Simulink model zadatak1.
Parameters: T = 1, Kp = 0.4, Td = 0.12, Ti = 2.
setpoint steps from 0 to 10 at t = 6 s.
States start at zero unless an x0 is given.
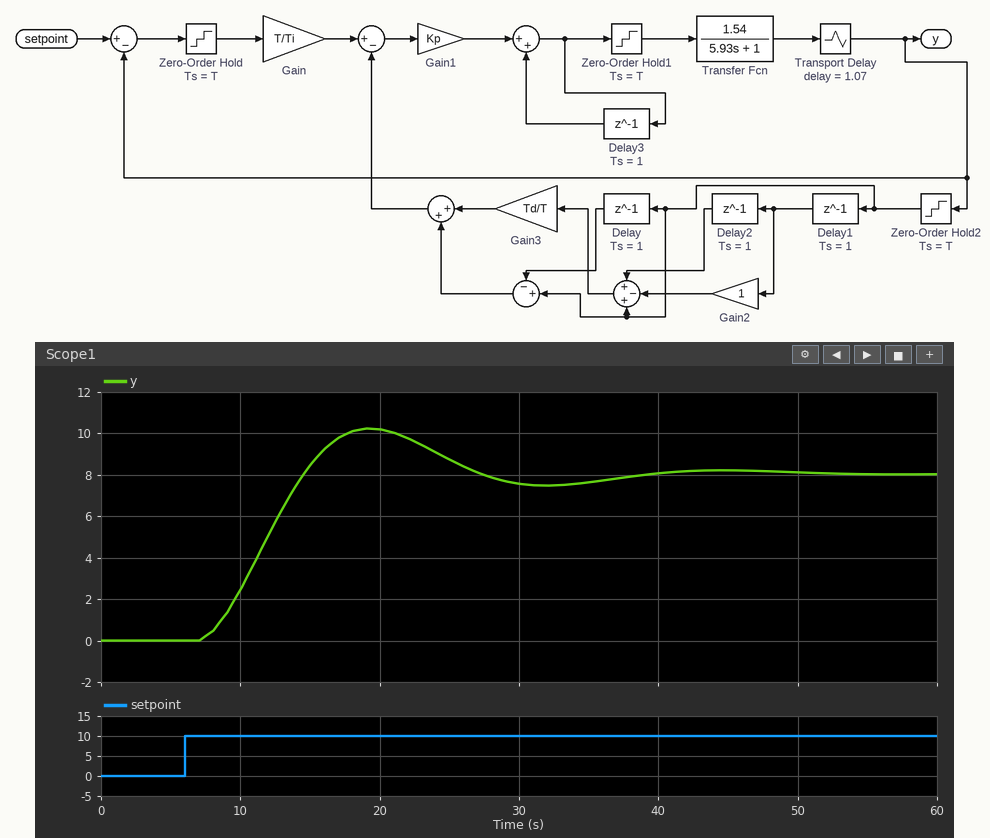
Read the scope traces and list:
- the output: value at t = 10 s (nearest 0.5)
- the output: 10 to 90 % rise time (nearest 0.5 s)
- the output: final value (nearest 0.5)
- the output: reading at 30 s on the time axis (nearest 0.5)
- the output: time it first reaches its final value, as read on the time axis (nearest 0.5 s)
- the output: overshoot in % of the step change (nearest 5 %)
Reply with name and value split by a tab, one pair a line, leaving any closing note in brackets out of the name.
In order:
the output: value at t = 10 s	2.5
the output: 10 to 90 % rise time	5.5 s
the output: final value	8.0
the output: reading at 30 s on the time axis	7.5
the output: time it first reaches its final value, as read on the time axis	14.5 s
the output: overshoot in % of the step change	25 %
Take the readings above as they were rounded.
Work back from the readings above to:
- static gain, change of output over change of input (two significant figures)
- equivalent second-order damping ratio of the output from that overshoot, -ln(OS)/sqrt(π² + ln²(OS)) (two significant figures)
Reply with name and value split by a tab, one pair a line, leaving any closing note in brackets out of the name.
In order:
static gain, change of output over change of input	0.80
equivalent second-order damping ratio of the output from that overshoot, -ln(OS)/sqrt(π² + ln²(OS))	0.40
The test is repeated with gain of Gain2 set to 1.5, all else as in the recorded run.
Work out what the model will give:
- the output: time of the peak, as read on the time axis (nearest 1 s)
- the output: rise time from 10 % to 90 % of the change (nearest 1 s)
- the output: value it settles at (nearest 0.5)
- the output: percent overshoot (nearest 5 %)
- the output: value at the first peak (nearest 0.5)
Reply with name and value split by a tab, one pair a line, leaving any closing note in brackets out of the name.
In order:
the output: time of the peak, as read on the time axis	20 s
the output: rise time from 10 % to 90 % of the change	6 s
the output: value it settles at	9.0
the output: percent overshoot	20 %
the output: value at the first peak	11.0
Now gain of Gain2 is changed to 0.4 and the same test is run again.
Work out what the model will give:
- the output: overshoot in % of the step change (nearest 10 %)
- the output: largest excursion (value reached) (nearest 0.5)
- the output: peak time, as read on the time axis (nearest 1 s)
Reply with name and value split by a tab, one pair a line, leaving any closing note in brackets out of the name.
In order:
the output: overshoot in % of the step change	30 %
the output: largest excursion (value reached)	9.5
the output: peak time, as read on the time axis	18 s
